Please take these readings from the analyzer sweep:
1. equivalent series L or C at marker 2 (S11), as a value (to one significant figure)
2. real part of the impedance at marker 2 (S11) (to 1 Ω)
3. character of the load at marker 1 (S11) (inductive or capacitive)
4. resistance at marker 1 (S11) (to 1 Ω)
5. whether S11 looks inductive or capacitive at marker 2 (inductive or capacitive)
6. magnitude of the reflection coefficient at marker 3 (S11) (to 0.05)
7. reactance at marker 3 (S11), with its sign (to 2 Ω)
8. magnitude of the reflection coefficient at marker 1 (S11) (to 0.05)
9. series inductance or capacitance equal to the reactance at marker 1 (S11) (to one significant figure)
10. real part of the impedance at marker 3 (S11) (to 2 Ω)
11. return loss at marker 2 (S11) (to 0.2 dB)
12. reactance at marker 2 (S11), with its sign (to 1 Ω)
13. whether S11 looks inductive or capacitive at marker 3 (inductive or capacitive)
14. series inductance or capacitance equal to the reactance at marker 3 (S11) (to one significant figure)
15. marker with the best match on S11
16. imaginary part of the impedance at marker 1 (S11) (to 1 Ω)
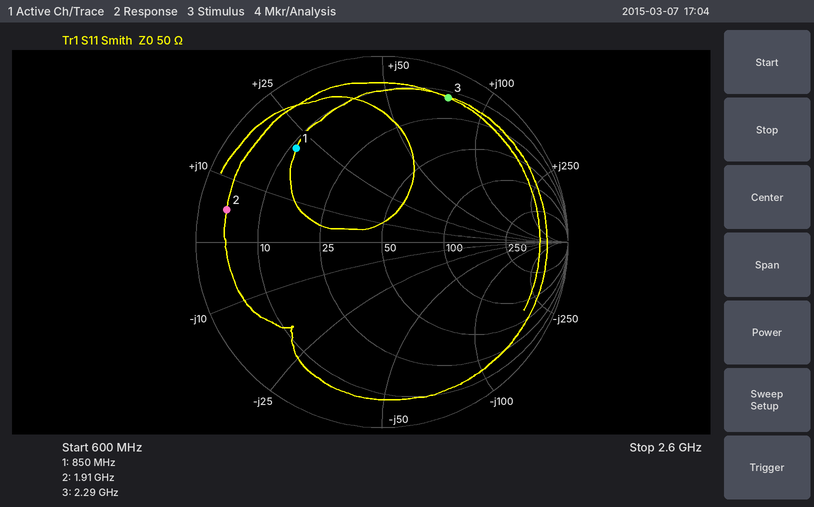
400 pH
4 Ω
inductive
11 Ω
inductive
0.85
+76 Ω
0.70
4 nH
14 Ω
1.4 dB
+5 Ω
inductive
5 nH
marker 1
+21 Ω
